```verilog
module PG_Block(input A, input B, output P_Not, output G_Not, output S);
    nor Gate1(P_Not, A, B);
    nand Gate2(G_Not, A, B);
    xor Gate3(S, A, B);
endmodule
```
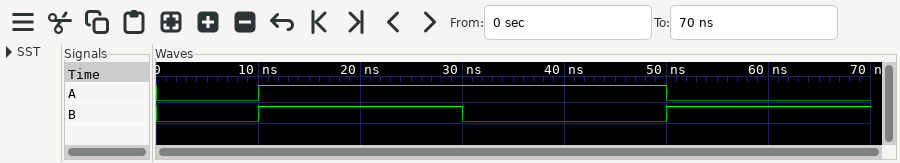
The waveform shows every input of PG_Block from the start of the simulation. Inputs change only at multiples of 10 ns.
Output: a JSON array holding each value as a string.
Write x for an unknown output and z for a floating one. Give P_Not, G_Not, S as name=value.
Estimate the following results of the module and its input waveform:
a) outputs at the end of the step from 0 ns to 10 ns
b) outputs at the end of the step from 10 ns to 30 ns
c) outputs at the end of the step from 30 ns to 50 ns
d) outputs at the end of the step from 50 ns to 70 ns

["P_Not=1, G_Not=1, S=0", "P_Not=0, G_Not=0, S=0", "P_Not=0, G_Not=1, S=1", "P_Not=0, G_Not=1, S=1"]
